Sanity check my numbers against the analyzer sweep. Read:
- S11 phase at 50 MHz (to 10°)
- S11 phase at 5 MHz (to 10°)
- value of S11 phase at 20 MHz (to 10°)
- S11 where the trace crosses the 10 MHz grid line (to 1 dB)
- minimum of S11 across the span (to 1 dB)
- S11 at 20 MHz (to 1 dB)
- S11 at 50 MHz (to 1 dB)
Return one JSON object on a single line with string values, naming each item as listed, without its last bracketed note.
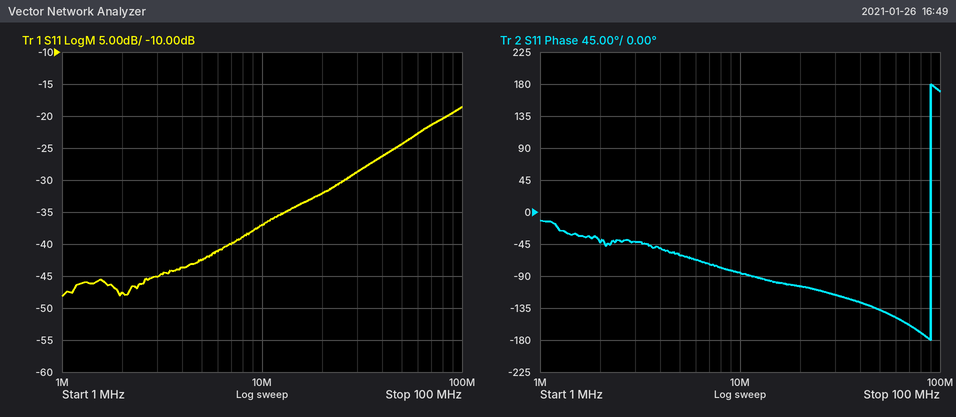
{"S11 phase at 50 MHz": "-140°", "S11 phase at 5 MHz": "-60°", "value of S11 phase at 20 MHz": "-100°", "S11 where the trace crosses the 10 MHz grid line": "-37 dB", "minimum of S11 across the span": "-48 dB", "S11 at 20 MHz": "-32 dB", "S11 at 50 MHz": "-24 dB"}
